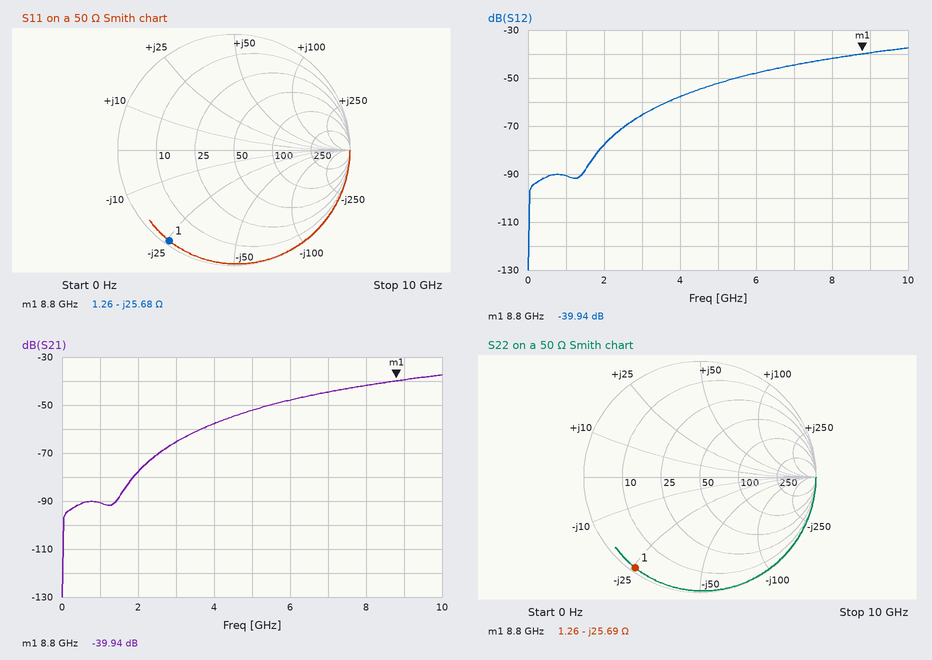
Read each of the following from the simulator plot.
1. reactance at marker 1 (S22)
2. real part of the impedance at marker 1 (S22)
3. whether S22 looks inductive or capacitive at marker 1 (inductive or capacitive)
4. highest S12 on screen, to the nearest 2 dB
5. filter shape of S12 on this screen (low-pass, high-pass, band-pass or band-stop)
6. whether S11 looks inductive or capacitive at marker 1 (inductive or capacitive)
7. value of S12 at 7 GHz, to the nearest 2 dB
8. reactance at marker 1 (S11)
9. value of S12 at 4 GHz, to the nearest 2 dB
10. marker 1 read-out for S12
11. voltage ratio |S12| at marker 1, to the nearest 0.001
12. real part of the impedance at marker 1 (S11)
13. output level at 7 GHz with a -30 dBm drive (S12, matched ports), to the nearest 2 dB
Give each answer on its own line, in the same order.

-25.69 Ω
1.26 Ω
capacitive
-38 dB
high-pass
capacitive
-44 dB
-25.68 Ω
-58 dB
-39.94 dB
0.010
1.26 Ω
-74 dBm
